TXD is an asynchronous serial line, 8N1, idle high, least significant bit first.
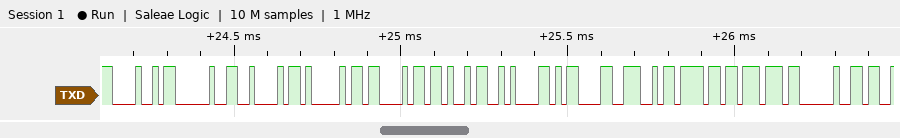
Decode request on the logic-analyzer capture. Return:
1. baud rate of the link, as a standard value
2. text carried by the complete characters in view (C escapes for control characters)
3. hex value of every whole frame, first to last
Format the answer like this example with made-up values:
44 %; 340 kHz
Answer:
57600 baud; "H BACK\n\rNow "; 0x48 0x20 0x42 0x41 0x43 0x4B 0x0A 0x0D 0x4E 0x6F 0x77 0x20
